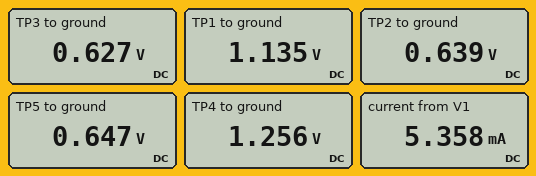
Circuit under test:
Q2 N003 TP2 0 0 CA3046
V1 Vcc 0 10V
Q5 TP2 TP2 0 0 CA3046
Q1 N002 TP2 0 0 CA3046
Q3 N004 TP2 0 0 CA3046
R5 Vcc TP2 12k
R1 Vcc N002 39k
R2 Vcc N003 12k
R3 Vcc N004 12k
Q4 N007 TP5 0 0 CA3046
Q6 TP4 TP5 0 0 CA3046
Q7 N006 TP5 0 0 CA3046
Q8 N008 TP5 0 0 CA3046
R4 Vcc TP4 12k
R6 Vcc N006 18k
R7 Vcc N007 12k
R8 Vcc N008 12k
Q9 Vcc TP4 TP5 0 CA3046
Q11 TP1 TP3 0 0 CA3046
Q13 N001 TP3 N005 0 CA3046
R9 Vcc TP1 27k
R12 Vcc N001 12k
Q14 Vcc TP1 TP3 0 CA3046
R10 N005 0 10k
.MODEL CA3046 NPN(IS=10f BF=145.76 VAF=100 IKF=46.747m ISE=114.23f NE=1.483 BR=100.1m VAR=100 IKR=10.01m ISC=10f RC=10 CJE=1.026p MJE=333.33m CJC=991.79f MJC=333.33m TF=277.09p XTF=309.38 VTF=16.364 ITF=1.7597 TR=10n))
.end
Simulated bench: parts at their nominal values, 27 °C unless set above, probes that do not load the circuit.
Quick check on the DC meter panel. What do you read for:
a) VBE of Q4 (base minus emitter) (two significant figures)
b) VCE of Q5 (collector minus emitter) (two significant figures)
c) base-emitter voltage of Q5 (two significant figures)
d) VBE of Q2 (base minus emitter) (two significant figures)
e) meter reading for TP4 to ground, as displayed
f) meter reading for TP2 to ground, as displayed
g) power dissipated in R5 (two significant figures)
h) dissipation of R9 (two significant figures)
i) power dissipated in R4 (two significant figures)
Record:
650 mV
640 mV
640 mV
640 mV
1.256 V
0.639 V
7.3 mW
2.9 mW
6.4 mW
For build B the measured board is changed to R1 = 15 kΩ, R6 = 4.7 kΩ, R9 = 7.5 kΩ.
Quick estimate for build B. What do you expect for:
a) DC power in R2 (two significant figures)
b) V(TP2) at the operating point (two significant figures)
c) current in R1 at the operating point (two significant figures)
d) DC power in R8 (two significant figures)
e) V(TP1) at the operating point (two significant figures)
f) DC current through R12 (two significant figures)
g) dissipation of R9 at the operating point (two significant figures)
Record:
6.1 mW
650 mV
660 µA
6.4 mW
1.2 V
12 µA
10 mW
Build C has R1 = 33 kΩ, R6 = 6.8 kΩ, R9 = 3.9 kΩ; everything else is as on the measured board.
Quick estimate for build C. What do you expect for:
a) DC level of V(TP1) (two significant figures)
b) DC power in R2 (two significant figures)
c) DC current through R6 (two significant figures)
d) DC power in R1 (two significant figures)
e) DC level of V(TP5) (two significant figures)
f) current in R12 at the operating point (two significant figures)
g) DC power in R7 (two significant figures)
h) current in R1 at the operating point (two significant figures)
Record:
1.2 V
3.7 mW
760 µA
3.0 mW
650 mV
13 µA
6.4 mW
300 µA
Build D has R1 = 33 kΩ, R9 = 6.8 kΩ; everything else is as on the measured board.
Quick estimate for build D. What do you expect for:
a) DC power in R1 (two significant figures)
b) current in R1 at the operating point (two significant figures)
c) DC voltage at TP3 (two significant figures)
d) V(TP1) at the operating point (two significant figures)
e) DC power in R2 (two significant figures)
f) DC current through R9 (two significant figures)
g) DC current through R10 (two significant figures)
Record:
3.0 mW
300 µA
660 mV
1.2 V
3.7 mW
1.3 mA
12 µA
